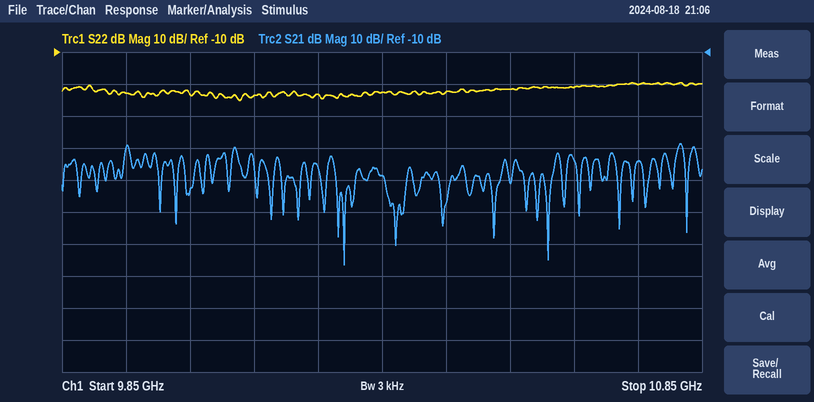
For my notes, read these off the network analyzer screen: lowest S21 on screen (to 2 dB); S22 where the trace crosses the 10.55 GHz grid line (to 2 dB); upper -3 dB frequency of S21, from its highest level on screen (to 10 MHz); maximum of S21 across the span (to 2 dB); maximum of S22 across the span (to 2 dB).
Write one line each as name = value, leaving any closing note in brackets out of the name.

lowest S21 on screen = -76 dB
S22 where the trace crosses the 10.55 GHz grid line = -22 dB
upper -3 dB frequency of S21, from its highest level on screen = 10.82 GHz
maximum of S21 across the span = -38 dB
maximum of S22 across the span = -20 dB
